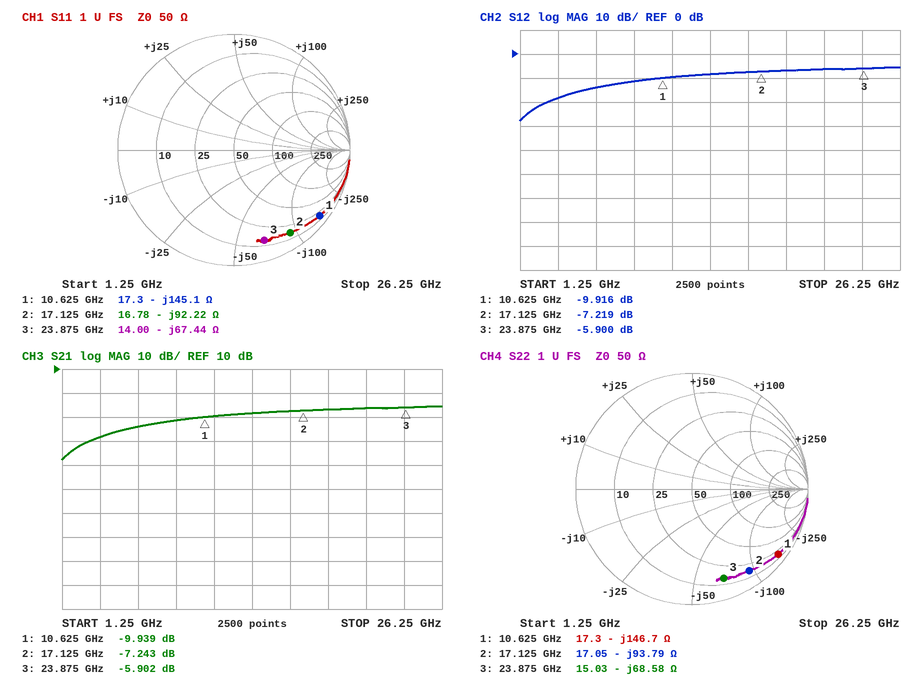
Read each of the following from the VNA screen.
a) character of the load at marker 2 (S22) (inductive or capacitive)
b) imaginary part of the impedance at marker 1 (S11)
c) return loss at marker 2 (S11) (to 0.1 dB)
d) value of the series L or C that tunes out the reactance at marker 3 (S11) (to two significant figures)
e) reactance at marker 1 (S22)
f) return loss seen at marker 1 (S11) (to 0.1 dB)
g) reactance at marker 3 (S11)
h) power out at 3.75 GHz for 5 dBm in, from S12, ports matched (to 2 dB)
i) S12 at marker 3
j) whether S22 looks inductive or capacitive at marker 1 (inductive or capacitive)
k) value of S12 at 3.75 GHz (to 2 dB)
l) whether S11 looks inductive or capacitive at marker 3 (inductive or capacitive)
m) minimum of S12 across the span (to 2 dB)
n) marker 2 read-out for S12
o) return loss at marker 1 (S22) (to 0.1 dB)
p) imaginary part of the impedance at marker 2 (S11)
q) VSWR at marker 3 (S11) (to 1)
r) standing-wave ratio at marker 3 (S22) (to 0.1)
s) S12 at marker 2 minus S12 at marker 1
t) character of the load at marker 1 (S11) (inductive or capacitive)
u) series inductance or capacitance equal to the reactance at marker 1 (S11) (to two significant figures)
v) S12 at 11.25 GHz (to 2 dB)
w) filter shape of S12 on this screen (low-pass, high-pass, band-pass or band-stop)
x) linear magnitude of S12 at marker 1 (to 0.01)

capacitive
-145.1 Ω
1.3 dB
450 pH
-146.7 Ω
0.6 dB
-67.44 Ω
-14 dBm
-5.900 dB
capacitive
-18 dB
capacitive
-28 dB
-7.219 dB
0.6 dB
-92.22 Ω
10
9.8
2.697 dB
capacitive
100 fF
-10 dB
high-pass
0.32
